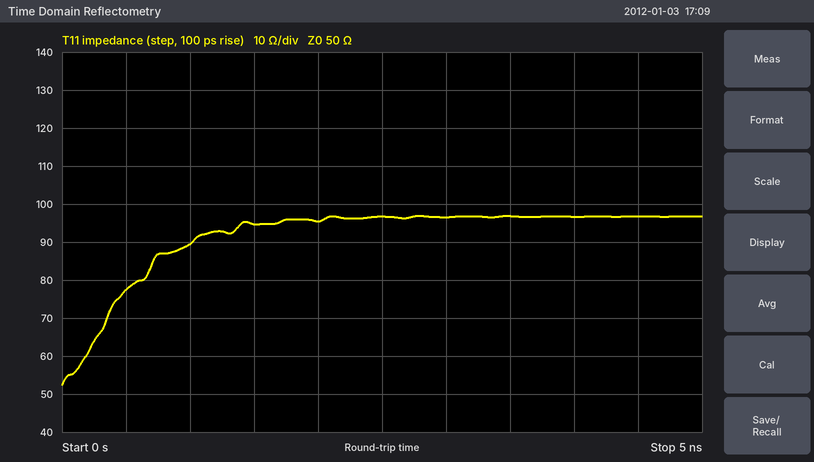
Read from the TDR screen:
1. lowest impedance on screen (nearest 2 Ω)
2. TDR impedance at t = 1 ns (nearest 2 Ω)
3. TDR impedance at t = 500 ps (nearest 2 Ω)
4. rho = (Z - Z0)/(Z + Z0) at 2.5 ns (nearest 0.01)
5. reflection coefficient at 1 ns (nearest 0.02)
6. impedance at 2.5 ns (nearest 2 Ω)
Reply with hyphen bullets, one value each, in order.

- 52 Ω
- 90 Ω
- 78 Ω
- +0.32
- +0.28
- 96 Ω
